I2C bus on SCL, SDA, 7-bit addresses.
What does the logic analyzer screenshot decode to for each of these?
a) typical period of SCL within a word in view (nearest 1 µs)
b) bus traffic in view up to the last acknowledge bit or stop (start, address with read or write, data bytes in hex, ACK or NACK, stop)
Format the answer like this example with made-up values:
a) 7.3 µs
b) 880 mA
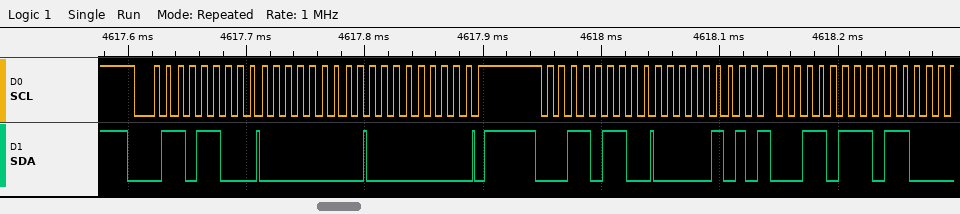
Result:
a) 10 µs
b) start, address 36 write ACK, 00 ACK, 00 ACK, stop, start, address 1B write ACK, 05 ACK, repeated start, address 1B read ACK
